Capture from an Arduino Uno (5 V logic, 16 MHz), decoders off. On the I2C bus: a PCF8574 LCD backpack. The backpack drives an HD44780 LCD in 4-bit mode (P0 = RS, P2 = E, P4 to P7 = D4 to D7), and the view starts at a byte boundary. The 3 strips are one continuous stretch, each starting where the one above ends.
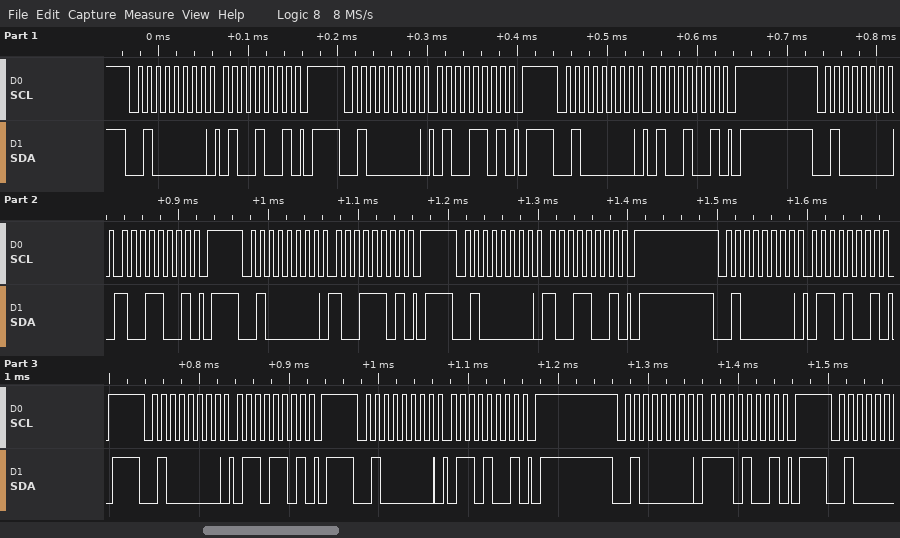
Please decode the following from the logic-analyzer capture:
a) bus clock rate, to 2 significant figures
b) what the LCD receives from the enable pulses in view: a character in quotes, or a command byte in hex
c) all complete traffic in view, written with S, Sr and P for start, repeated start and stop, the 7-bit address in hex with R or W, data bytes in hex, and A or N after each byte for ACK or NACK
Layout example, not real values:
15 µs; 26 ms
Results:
100 kHz; 'I'; S 20W A 49 A P S 20W A 4D A P S 20W A 49 A P S 20W A 99 A P S 20W A 9D A P S 20W A 99 A P S 20W A 69 A P S 20W A 6D A P S 20W A 69 A P S 20W A E9 A P
